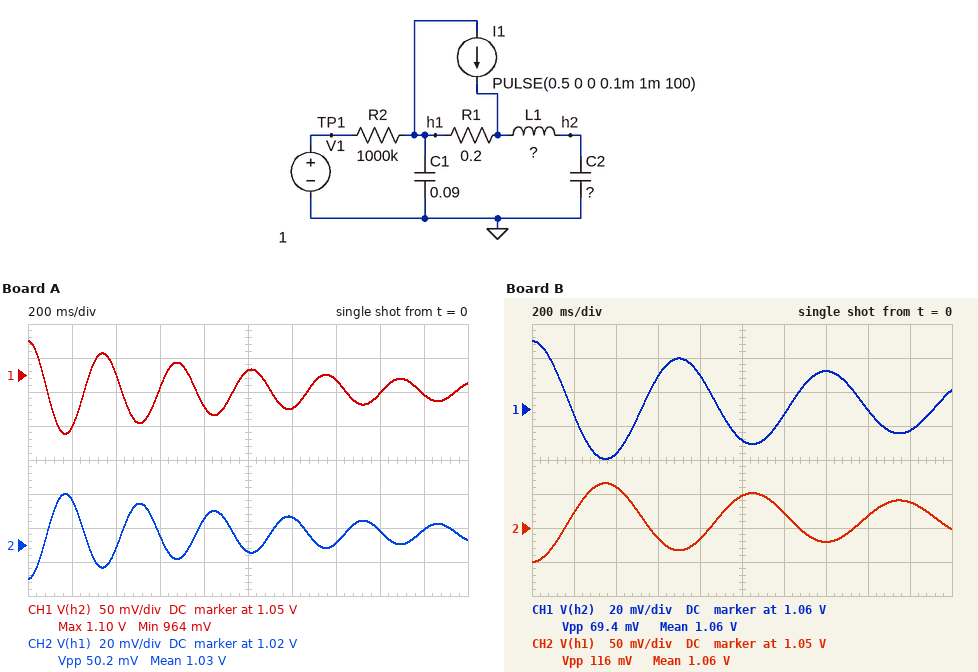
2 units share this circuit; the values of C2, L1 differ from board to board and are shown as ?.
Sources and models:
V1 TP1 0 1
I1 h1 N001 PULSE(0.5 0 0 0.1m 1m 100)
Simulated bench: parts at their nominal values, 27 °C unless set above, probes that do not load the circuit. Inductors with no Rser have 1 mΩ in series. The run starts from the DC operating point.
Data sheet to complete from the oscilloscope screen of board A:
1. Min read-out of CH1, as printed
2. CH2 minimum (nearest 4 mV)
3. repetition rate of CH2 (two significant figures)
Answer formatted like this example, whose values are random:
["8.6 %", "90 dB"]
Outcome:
["964 mV", "1.000 V", "3.0 Hz"]
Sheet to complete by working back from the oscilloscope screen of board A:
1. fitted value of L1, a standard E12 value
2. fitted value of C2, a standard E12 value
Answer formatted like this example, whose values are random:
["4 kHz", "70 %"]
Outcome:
["120 mH", "33 mF"]
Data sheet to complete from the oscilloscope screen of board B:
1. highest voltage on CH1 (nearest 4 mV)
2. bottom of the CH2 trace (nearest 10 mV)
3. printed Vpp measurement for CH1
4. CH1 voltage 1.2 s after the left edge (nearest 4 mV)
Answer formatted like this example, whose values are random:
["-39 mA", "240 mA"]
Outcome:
["1.100 V", "1.00 V", "69.4 mV", "1.056 V"]
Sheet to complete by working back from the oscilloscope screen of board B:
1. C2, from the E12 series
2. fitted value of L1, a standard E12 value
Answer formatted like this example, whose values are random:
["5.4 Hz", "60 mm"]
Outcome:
["150 mF", "220 mH"]
